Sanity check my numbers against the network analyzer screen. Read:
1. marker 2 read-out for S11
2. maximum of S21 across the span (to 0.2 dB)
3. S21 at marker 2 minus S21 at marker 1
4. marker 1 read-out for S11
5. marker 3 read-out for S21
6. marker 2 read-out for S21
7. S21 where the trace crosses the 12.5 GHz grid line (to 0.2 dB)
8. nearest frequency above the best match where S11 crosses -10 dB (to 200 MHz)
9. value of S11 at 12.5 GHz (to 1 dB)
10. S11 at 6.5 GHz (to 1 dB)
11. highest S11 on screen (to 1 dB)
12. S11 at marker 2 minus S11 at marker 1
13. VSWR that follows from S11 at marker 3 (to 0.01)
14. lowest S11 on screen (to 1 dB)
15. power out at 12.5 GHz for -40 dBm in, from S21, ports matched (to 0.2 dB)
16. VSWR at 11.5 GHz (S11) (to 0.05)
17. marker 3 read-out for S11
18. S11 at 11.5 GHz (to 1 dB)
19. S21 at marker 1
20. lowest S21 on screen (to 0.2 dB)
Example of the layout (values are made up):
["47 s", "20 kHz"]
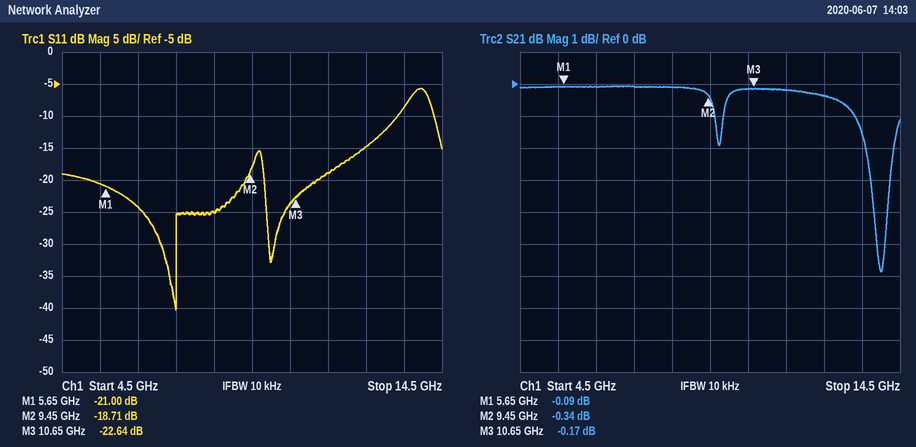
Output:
["-18.71 dB", "0.0 dB", "-0.25 dB", "-21.00 dB", "-0.17 dB", "-0.34 dB", "-0.4 dB", "13.4 GHz", "-15 dB", "-24 dB", "-6 dB", "2.29 dB", "1.16", "-40 dB", "-40.4 dBm", "1.25", "-22.64 dB", "-19 dB", "-0.09 dB", "-5.8 dB"]
